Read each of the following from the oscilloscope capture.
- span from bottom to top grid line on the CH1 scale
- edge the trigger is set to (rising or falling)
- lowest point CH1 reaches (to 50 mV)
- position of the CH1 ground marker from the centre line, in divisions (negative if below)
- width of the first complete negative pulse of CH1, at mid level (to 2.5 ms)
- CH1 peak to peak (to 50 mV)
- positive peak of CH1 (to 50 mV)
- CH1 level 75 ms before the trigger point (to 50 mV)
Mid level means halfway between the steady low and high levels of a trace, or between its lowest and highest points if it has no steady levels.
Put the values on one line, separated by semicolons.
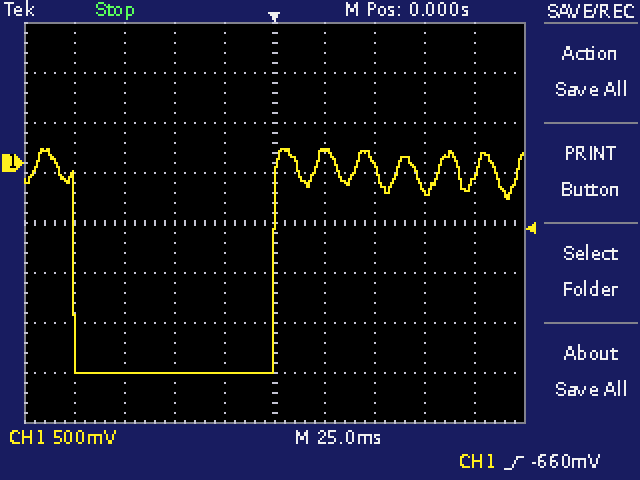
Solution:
4 V; rising; -2.10 V; +1.2 div; 100.0 ms; 2.25 V; 150 mV; -2.10 V
